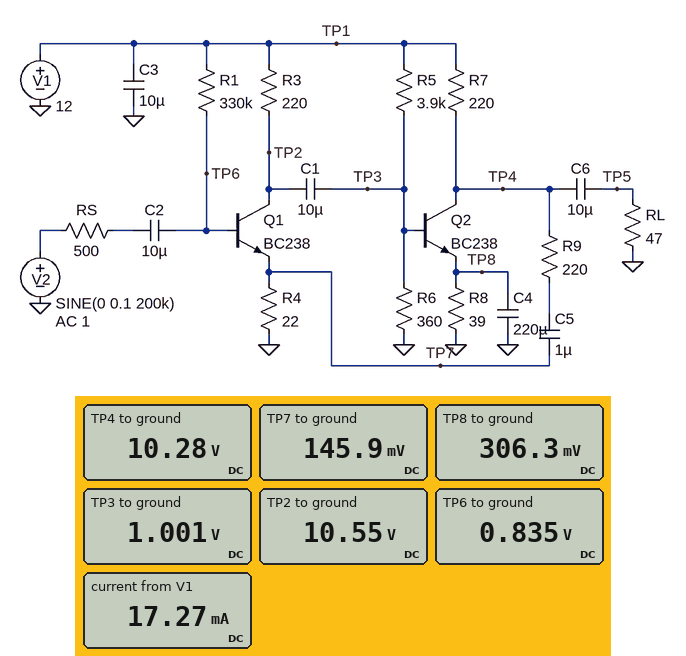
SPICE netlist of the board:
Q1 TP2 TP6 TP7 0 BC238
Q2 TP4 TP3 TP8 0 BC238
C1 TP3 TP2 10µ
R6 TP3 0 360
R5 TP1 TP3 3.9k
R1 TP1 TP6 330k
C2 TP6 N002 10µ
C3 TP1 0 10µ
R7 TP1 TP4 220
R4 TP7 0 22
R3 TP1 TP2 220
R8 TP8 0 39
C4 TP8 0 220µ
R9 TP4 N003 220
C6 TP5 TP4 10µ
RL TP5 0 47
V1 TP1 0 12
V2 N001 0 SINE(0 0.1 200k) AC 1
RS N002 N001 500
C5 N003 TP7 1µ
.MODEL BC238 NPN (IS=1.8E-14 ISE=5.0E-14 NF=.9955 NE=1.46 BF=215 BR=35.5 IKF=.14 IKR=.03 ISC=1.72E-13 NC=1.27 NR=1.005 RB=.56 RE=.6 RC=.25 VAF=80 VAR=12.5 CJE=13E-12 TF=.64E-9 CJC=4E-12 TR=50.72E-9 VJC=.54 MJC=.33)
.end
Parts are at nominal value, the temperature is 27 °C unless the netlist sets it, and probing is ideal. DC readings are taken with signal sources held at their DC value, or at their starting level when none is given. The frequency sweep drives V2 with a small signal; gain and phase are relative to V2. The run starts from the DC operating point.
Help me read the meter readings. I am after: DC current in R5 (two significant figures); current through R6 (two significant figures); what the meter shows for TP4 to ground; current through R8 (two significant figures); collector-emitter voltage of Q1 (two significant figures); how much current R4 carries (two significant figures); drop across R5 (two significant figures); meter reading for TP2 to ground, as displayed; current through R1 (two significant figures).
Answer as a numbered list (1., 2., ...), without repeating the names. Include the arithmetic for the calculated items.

1. (12 V - 1.001 V) / 3.9 kΩ = 2.8 mA
2. (1.001 V) / 360 Ω = 2.8 mA
3. 10.28 V
4. (306.3 mV) / 39 Ω = 7.9 mA
5. 10.55 V - 145.9 mV = 10 V
6. (145.9 mV) / 22 Ω = 6.6 mA
7. 12 V - 1.001 V = 11 V
8. 10.55 V
9. (12 V - 835 mV) / 330 kΩ = 34 µA
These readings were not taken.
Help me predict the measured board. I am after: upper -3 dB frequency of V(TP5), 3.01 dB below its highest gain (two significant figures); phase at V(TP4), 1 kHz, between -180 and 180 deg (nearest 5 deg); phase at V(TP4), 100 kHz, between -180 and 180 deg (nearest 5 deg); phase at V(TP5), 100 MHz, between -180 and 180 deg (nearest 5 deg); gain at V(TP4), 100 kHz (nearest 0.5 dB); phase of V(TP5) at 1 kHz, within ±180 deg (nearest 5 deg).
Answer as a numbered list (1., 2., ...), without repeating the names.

1. 790 Hz
2. -25 deg
3. 0 deg
4. -170 deg
5. 18.5 dB
6. -5 deg
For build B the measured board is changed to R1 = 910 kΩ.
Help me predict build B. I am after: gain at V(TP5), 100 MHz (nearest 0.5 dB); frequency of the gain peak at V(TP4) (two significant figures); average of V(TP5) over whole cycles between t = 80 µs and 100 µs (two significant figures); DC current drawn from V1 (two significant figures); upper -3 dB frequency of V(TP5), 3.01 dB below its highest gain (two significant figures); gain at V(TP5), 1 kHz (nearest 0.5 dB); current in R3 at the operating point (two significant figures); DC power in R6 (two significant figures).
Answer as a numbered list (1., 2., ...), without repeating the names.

1. -13.0 dB
2. 74 Hz
3. -170 mV
4. 13 mA
5. 1.0 kHz
6. 19.0 dB
7. 2.4 mA
8. 2.8 mW
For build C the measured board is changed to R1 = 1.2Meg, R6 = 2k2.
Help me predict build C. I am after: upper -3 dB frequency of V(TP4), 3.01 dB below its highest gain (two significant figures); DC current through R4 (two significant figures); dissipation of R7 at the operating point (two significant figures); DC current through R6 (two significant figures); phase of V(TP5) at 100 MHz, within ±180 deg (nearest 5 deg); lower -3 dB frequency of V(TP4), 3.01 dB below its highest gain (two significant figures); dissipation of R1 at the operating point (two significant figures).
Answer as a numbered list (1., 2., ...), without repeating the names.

1. 220 kHz
2. 1.8 mA
3. 460 mW
4. 1.2 mA
5. 80 deg
6. 78 Hz
7. 110 µW
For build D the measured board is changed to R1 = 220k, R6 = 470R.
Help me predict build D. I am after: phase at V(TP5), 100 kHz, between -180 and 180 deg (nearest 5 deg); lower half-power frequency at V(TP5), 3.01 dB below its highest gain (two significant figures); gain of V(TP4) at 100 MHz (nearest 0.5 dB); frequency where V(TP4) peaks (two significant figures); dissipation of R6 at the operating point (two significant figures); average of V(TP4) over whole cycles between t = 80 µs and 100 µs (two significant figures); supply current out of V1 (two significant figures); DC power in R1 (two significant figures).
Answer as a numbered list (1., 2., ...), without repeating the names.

1. 0 deg
2. 60 Hz
3. -10.5 dB
4. 68 Hz
5. 3.4 mW
6. 8.8 V
7. 26 mA
8. 560 µW
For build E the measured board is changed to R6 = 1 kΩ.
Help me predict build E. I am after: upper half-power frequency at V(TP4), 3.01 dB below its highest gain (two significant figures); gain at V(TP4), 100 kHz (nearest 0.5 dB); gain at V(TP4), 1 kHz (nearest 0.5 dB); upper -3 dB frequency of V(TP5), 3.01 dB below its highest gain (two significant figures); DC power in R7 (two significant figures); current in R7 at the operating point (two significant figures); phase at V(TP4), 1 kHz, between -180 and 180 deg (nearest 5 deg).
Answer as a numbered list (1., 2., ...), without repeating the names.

1. 120 Hz
2. 19.5 dB
3. 21.0 dB
4. 570 Hz
5. 320 mW
6. 38 mA
7. -30 deg
